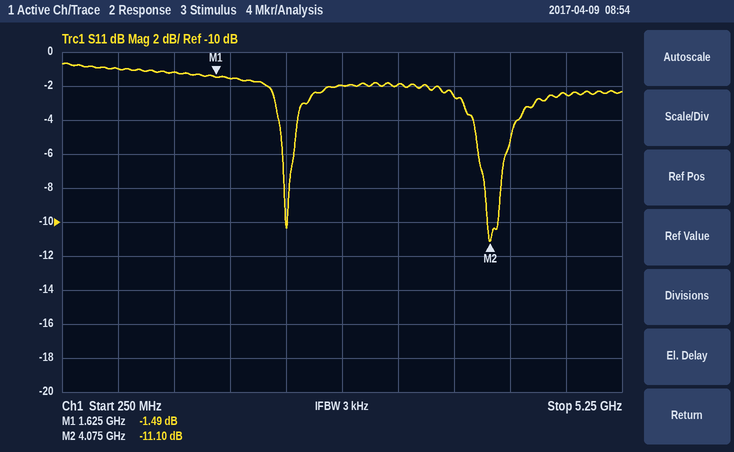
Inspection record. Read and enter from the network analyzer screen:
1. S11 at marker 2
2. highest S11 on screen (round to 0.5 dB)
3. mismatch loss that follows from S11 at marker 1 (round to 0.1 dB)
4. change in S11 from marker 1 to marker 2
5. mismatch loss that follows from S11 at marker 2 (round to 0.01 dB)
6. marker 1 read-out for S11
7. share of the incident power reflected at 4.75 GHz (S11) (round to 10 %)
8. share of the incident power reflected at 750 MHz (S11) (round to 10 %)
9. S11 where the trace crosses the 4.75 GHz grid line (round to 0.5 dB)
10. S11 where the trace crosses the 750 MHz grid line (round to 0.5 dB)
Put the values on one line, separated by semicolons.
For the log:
-11.10 dB; -0.5 dB; 5.4 dB; -9.61 dB; 0.35 dB; -1.49 dB; 60 %; 80 %; -2.5 dB; -1.0 dB
